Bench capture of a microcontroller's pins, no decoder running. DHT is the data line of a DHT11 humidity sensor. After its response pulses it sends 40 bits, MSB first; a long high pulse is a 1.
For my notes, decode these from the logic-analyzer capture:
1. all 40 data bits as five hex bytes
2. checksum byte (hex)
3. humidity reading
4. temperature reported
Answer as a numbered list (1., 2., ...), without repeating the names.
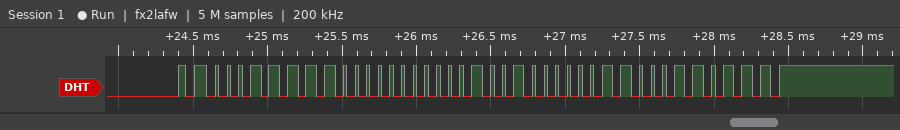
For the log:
1. 1F 00 12 06 37
2. 0x37
3. 31 %
4. 18.6 °C
